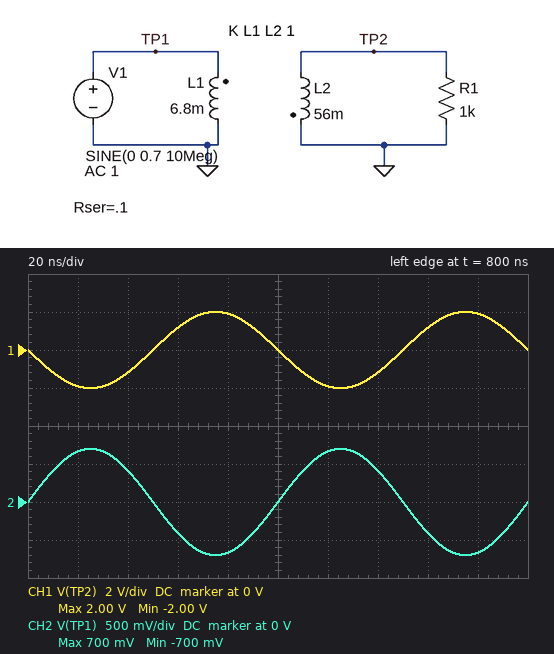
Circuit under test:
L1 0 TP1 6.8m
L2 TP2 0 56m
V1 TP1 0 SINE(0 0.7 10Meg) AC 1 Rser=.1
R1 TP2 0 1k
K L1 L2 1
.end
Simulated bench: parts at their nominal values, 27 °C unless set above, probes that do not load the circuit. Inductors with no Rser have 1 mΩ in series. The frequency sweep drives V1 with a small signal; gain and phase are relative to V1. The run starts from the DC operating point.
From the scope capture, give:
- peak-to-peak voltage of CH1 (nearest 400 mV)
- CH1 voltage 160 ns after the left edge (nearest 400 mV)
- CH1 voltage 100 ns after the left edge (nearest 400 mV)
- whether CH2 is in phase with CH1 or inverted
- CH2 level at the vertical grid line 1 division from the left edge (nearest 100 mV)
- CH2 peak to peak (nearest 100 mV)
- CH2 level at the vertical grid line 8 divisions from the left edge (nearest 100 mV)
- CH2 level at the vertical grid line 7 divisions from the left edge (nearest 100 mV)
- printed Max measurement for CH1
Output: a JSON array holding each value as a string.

["4.0 V", "1.2 V", "0 V", "inverted", "700 mV", "1.4 V", "-400 mV", "400 mV", "2.00 V"]
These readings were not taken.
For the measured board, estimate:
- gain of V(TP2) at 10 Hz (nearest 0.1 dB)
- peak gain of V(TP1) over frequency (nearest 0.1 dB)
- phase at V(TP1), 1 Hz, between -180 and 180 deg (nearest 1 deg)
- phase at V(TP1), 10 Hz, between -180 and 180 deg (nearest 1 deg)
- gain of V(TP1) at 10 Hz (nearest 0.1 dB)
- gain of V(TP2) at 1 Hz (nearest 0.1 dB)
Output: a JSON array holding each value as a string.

["8.9 dB", "0 dB", "66 deg", "13 deg", "-0.2 dB", "1.0 dB"]
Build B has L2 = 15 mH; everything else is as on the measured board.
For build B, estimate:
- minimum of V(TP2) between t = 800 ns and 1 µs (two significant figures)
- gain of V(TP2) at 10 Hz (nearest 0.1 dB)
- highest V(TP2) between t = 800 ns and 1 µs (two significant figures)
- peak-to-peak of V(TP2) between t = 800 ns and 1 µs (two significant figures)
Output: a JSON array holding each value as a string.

["-1.0 V", "3.2 dB", "1.0 V", "2.1 V"]
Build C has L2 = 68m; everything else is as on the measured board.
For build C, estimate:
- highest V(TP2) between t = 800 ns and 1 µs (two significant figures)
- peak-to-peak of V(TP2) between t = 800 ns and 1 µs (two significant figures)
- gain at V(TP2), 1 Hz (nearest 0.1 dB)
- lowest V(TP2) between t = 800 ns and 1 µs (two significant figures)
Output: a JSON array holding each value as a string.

["2.2 V", "4.4 V", "1.8 dB", "-2.2 V"]
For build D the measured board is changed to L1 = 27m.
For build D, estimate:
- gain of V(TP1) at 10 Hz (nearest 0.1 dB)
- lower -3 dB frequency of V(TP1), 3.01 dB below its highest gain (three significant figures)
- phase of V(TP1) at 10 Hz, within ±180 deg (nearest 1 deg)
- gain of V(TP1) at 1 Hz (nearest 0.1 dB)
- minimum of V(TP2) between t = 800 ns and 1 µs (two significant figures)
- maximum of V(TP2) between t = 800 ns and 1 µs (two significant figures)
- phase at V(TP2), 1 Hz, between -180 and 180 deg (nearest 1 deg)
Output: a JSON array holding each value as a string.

["0 dB", "595 mHz", "3 deg", "-1.3 dB", "-1.0 V", "1.0 V", "-149 deg"]
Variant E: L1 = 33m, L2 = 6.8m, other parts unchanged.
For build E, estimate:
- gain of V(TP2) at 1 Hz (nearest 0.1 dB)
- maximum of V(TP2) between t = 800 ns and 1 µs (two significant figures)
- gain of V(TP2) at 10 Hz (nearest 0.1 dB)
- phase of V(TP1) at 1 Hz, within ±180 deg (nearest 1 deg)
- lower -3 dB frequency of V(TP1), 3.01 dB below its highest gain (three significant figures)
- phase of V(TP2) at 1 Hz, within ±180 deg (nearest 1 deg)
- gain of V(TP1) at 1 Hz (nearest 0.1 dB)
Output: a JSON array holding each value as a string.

["-7.8 dB", "320 mV", "-6.9 dB", "26 deg", "487 mHz", "-154 deg", "-0.9 dB"]
